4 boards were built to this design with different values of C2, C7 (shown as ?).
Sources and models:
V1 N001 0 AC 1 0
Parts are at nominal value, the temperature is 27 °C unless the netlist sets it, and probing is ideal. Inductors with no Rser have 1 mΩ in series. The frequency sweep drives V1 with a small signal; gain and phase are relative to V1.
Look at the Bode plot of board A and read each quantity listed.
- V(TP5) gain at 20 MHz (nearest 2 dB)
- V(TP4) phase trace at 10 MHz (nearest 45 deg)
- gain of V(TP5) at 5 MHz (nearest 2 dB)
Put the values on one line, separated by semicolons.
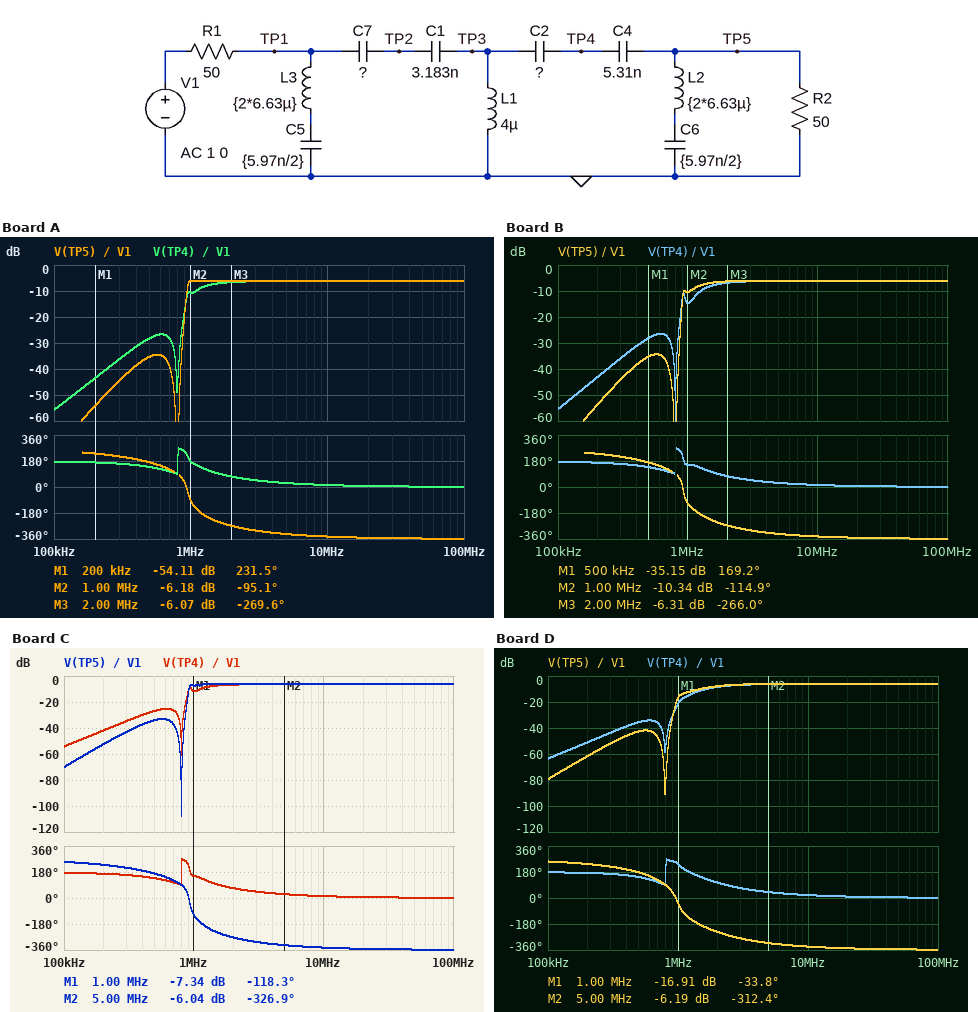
-6 dB; 0 deg; -6 dB
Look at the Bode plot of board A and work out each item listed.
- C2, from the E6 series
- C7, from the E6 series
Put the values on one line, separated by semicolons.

4.7 nF; 6.8 nF
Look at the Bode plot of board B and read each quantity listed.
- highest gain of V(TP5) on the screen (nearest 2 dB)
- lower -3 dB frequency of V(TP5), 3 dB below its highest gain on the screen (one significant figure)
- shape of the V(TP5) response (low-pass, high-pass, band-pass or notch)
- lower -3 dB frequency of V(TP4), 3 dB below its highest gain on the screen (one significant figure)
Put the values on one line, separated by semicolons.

-6 dB; 1 MHz; high-pass; 1 MHz
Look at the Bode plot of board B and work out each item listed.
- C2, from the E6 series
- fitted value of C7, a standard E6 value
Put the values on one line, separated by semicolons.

10 nF; 3.3 nF
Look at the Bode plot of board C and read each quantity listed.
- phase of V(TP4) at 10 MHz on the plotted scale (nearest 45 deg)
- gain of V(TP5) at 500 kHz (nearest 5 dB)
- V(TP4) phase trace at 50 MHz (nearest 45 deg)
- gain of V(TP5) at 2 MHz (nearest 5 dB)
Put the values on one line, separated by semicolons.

0 deg; -35 dB; 0 deg; -5 dB
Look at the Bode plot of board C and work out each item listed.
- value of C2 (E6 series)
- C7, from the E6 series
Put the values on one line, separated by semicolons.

6.8 nF; 6.8 nF
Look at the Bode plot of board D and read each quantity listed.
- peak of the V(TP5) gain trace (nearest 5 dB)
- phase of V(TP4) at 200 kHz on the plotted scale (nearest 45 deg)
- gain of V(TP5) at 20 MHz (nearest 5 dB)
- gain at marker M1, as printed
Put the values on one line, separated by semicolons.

-5 dB; 180 deg; -5 dB; -16.91 dB
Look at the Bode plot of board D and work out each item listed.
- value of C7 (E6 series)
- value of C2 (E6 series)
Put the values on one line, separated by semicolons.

15 nF; 1 nF
